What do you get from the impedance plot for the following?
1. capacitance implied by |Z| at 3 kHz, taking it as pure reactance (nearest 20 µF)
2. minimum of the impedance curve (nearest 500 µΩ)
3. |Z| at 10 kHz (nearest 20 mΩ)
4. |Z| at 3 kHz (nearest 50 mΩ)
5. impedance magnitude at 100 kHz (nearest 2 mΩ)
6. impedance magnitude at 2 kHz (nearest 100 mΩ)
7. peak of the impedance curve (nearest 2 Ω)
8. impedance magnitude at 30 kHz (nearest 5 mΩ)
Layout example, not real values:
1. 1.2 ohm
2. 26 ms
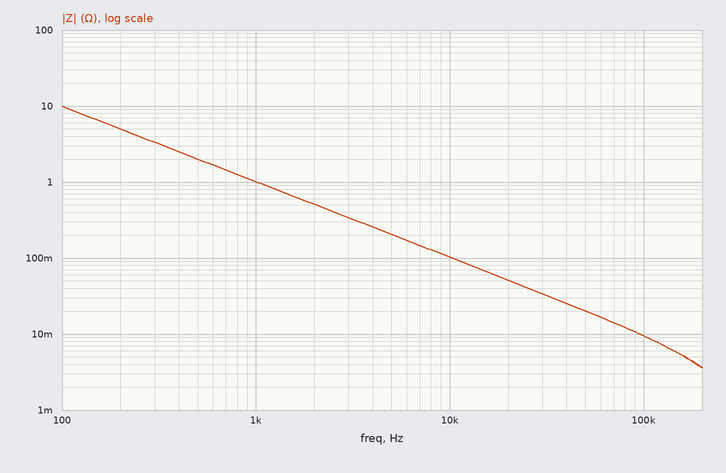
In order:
1. 160 µF
2. 3.5 mΩ
3. 100 mΩ
4. 350 mΩ
5. 10 mΩ
6. 500 mΩ
7. 10 Ω
8. 35 mΩ
